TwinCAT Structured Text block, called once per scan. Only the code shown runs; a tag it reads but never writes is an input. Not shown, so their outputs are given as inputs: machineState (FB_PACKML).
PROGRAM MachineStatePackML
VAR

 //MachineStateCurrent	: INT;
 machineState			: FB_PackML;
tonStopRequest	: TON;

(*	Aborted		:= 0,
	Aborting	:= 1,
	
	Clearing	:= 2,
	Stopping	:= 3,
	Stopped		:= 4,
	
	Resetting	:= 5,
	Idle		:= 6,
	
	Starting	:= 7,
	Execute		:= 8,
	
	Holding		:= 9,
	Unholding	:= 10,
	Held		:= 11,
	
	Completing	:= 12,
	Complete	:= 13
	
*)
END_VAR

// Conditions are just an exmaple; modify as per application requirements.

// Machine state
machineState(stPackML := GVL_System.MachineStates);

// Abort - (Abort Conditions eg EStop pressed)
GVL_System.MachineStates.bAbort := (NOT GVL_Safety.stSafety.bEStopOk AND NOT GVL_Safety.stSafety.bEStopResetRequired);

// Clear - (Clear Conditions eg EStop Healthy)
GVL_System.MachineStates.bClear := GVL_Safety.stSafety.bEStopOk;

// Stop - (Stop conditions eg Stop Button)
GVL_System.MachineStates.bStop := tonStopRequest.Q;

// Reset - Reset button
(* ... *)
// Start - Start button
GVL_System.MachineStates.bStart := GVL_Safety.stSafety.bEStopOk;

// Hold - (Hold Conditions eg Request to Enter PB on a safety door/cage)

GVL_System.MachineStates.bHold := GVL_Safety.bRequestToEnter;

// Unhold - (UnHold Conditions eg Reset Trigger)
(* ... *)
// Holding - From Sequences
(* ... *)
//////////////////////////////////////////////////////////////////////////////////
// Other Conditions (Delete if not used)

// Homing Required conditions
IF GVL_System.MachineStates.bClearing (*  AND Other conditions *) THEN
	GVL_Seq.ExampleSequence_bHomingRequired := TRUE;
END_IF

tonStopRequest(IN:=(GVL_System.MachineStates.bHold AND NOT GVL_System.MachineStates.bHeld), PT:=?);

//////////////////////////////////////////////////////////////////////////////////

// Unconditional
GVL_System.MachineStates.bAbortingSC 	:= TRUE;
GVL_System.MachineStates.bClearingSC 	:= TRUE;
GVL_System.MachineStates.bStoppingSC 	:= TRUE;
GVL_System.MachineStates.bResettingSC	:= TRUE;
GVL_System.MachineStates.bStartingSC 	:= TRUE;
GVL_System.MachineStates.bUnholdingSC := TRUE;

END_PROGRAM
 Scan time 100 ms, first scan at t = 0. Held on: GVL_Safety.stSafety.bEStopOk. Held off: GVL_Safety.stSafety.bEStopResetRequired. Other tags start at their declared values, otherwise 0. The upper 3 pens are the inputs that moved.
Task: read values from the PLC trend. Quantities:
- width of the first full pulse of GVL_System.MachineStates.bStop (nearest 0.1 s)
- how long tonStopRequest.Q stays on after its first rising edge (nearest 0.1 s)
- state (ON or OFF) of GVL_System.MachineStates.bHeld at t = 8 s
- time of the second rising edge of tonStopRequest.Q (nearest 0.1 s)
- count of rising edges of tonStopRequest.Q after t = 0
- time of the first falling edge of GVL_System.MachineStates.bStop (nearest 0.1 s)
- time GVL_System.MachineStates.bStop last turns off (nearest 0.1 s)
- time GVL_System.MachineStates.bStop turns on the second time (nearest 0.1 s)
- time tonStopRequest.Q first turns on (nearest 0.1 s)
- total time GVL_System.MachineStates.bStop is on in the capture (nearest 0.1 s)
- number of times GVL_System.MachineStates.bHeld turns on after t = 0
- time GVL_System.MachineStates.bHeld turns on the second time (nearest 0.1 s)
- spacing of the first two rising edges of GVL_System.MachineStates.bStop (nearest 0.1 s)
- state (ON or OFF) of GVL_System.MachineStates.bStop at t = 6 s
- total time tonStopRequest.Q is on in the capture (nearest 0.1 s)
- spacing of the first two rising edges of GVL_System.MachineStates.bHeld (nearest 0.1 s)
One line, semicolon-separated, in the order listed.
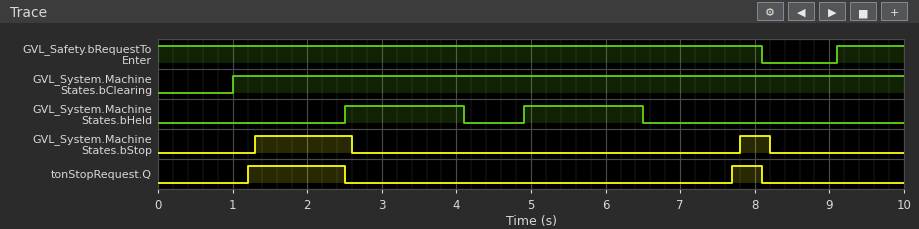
1.3 s; 1.3 s; OFF; 7.7 s; 2; 2.6 s; 8.2 s; 7.8 s; 1.2 s; 1.7 s; 2; 4.9 s; 6.5 s; OFF; 1.7 s; 2.4 s
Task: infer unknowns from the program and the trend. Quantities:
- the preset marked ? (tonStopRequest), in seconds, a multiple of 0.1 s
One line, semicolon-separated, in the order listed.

1.2 s
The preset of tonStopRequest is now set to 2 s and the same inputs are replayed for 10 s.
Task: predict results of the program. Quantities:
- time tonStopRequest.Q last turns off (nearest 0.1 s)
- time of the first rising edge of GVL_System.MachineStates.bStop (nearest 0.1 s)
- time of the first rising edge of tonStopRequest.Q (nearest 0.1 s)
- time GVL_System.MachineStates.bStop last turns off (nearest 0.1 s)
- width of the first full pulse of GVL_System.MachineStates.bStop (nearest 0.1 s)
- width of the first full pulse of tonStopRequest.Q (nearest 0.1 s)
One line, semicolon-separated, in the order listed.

2.5 s; 2.1 s; 2.0 s; 2.6 s; 0.5 s; 0.5 s
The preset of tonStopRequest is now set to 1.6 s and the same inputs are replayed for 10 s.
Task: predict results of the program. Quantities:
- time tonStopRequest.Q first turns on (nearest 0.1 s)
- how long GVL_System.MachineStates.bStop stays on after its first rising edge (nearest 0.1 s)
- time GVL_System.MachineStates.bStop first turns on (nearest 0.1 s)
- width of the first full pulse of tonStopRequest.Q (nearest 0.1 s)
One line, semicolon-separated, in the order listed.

1.6 s; 0.9 s; 1.7 s; 0.9 s
